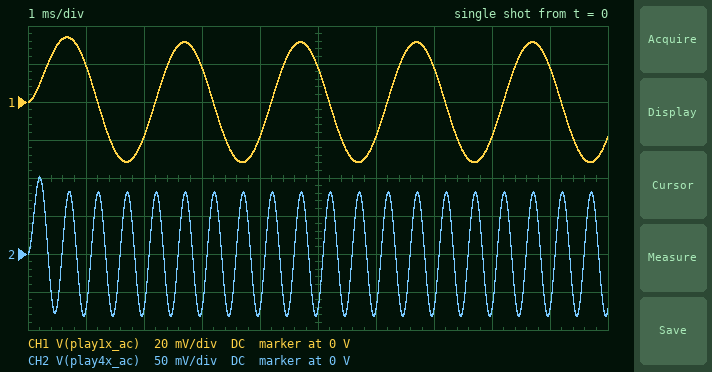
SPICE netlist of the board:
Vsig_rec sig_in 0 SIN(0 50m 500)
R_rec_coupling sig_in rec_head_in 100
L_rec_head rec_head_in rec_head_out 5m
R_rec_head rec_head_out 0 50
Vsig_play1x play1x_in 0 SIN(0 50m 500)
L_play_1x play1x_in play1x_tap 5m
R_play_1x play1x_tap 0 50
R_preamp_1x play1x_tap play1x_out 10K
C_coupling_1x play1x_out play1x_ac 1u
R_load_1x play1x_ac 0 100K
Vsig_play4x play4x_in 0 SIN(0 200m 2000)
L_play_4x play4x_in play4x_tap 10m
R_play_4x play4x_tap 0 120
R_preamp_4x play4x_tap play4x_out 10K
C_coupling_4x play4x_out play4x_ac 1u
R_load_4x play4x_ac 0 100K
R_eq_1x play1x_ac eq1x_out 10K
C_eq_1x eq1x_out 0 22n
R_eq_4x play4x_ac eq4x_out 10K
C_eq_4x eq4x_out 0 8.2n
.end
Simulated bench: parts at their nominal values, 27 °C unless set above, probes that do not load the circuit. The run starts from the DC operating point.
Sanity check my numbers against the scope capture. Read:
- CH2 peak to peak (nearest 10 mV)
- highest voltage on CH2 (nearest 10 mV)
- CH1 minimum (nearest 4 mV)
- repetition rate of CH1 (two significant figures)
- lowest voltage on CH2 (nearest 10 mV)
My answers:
180 mV
100 mV
-32 mV
500 Hz
-80 mV
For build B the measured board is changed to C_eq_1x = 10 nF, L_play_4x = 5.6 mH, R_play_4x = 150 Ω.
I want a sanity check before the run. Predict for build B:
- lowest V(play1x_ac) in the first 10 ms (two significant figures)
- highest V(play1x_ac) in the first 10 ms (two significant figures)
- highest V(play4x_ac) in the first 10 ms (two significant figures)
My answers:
-39 mV
39 mV
120 mV
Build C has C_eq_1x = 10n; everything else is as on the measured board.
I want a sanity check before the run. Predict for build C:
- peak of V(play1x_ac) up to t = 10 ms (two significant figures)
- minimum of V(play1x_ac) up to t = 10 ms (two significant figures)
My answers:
39 mV
-39 mV
